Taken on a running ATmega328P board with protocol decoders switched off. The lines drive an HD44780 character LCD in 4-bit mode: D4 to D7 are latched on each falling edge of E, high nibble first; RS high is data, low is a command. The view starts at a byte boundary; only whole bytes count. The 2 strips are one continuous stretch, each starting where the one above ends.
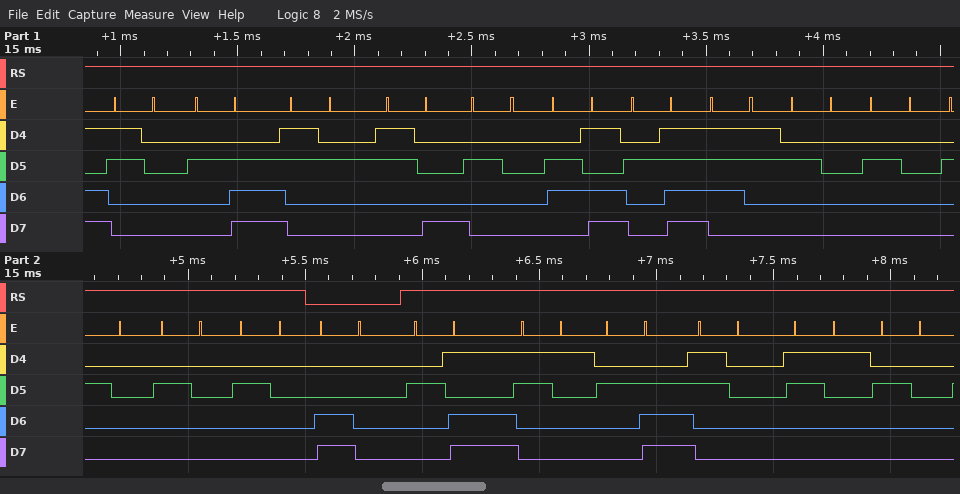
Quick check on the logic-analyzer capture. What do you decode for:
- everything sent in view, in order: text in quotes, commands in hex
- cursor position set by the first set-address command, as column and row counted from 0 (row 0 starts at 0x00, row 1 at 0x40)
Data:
"0.28 m/s     " 0xC0 "-1.01 "
column 0, row 1
